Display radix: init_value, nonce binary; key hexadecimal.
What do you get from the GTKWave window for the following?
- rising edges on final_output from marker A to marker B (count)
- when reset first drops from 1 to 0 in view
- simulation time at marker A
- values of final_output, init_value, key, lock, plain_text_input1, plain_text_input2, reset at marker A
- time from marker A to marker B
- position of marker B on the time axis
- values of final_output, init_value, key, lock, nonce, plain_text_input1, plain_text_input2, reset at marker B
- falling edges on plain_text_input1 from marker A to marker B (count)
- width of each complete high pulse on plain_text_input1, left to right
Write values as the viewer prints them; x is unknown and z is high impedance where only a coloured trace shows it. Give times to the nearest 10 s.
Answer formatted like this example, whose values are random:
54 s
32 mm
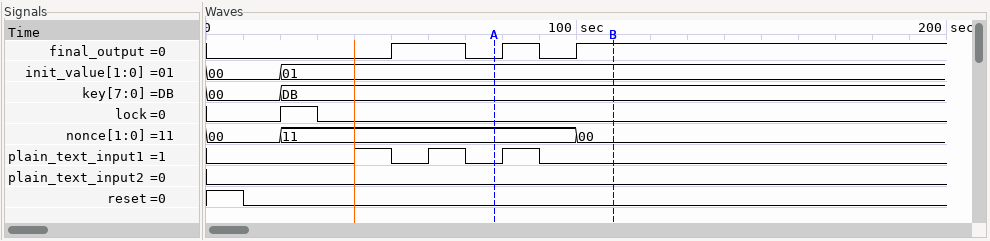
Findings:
2
10 s
80 s
final_output=0, init_value=01, key=DB, lock=0, plain_text_input1=0, plain_text_input2=0, reset=0
30 s
110 s
final_output=1, init_value=01, key=DB, lock=0, nonce=00, plain_text_input1=0, plain_text_input2=0, reset=0
1
10 s, 10 s, 10 s
